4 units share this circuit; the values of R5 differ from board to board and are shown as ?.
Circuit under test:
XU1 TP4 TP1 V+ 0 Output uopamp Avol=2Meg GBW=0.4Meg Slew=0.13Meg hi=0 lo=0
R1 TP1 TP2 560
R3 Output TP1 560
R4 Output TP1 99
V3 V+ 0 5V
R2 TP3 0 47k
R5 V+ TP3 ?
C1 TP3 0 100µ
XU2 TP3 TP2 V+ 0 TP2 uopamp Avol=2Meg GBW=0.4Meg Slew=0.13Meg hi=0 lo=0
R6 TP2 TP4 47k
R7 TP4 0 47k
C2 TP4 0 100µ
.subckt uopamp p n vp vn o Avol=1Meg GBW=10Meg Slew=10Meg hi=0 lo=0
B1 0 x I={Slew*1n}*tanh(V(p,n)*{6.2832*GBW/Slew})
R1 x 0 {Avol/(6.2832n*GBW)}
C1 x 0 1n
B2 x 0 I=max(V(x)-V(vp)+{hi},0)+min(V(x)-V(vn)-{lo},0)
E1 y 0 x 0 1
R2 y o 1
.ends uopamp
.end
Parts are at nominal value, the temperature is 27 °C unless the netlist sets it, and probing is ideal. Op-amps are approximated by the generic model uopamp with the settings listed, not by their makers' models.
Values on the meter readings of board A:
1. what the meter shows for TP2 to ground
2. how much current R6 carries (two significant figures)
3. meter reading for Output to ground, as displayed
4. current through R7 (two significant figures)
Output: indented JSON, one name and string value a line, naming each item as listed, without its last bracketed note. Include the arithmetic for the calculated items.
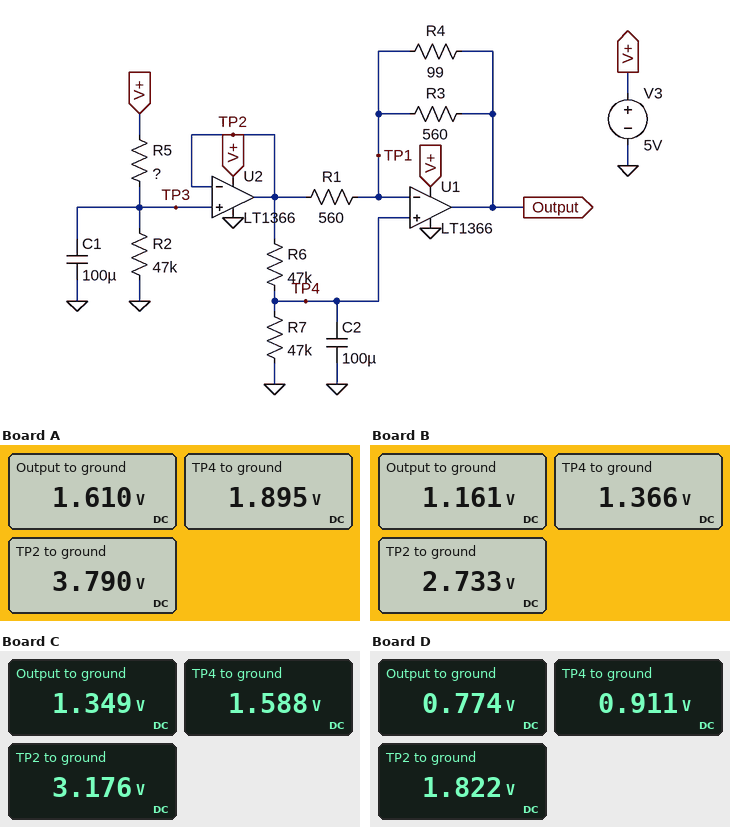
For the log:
{
  "what the meter shows for TP2 to ground": "3.790 V",
  "how much current R6 carries": "(3.79 V - 1.895 V) / 47 kΩ = 40 µA",
  "meter reading for Output to ground, as displayed": "1.610 V",
  "current through R7": "(1.895 V) / 47 kΩ = 40 µA"
}
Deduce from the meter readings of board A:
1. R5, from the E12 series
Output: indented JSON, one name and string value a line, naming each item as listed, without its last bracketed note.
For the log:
{
  "R5, from the E12 series": "15 kΩ"
}
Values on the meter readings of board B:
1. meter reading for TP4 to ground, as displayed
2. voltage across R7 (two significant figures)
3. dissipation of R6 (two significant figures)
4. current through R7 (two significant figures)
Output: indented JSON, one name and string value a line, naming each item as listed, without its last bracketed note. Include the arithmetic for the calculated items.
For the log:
{
  "meter reading for TP4 to ground, as displayed": "1.366 V",
  "voltage across R7": "1.366 V = 1.4 V",
  "dissipation of R6": "(2.733 V - 1.366 V)^2 / 47 kΩ = 40 µW",
  "current through R7": "(1.366 V) / 47 kΩ = 29 µA"
}
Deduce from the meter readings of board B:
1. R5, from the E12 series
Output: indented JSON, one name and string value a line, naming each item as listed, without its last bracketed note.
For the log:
{
  "R5, from the E12 series": "39 kΩ"
}
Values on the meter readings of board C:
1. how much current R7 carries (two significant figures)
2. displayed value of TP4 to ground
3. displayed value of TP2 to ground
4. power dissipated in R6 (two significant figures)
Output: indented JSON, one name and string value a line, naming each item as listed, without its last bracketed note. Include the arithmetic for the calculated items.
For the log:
{
  "how much current R7 carries": "(1.588 V) / 47 kΩ = 34 µA",
  "displayed value of TP4 to ground": "1.588 V",
  "displayed value of TP2 to ground": "3.176 V",
  "power dissipated in R6": "(3.176 V - 1.588 V)^2 / 47 kΩ = 54 µW"
}
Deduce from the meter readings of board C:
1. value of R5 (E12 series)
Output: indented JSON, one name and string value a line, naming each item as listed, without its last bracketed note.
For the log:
{
  "value of R5": "27 kΩ"
}
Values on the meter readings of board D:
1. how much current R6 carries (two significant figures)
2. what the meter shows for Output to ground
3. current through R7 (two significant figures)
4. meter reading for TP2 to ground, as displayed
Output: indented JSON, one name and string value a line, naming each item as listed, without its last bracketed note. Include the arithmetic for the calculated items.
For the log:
{
  "how much current R6 carries": "(1.822 V - 911 mV) / 47 kΩ = 19 µA",
  "what the meter shows for Output to ground": "0.774 V",
  "current through R7": "(911 mV) / 47 kΩ = 19 µA",
  "meter reading for TP2 to ground, as displayed": "1.822 V"
}
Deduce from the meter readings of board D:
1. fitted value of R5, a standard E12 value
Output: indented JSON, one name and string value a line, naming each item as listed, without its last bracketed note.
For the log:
{
  "fitted value of R5, a standard E12 value": "82 kΩ"
}
